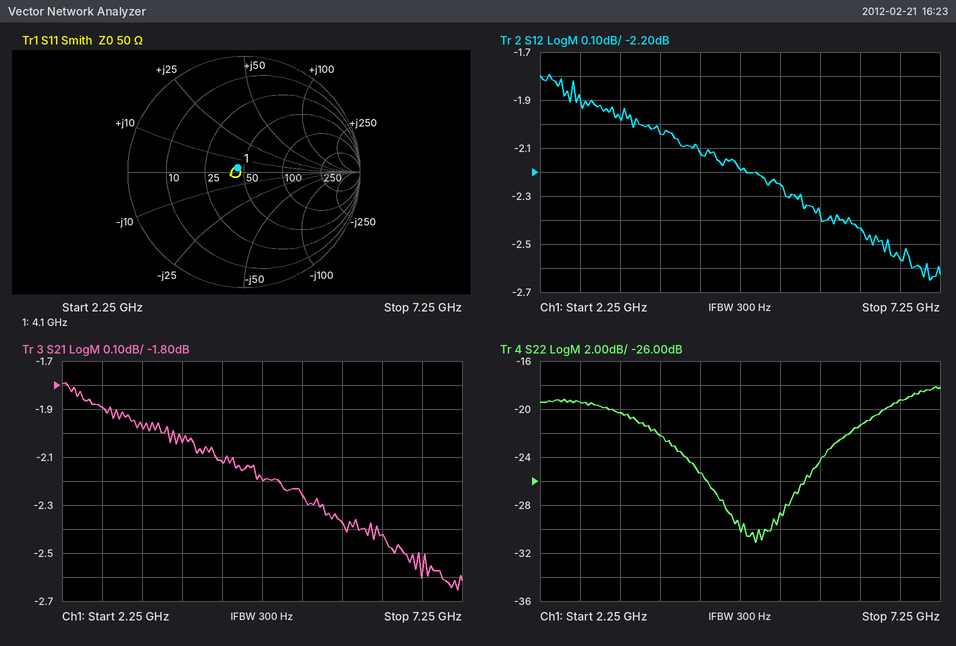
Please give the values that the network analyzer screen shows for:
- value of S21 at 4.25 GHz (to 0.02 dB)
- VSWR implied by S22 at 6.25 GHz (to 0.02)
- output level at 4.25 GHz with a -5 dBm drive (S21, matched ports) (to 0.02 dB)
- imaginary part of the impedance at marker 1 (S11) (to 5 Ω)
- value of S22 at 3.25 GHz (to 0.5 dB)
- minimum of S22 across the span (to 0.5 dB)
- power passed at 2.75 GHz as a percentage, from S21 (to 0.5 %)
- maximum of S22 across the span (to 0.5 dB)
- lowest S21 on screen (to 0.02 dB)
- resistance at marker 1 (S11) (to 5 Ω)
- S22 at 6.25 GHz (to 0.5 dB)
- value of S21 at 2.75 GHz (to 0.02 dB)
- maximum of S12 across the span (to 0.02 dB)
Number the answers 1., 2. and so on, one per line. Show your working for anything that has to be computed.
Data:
1. -2.12 dB
2. |Γ| = 10^(-21.5/20) = 0.0841; VSWR = (1 + 0.0841)/(1 − 0.0841) ≈ 1.18
3. -5 dBm + (-2.12 dB) = -7.12 dBm
4. +5 Ω
5. -20.5 dB
6. -31.0 dB
7. 10^(-1.9/10) ≈ 64.6 %, so 64.5 % to the nearest 0.5 %
8. -18.0 dB
9. -2.66 dB
10. 45 Ω
11. -21.5 dB
12. -1.90 dB
13. -1.80 dB
